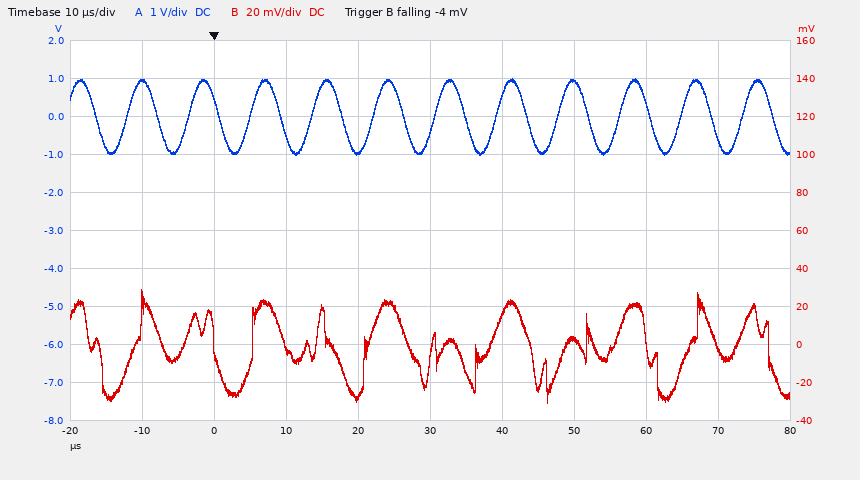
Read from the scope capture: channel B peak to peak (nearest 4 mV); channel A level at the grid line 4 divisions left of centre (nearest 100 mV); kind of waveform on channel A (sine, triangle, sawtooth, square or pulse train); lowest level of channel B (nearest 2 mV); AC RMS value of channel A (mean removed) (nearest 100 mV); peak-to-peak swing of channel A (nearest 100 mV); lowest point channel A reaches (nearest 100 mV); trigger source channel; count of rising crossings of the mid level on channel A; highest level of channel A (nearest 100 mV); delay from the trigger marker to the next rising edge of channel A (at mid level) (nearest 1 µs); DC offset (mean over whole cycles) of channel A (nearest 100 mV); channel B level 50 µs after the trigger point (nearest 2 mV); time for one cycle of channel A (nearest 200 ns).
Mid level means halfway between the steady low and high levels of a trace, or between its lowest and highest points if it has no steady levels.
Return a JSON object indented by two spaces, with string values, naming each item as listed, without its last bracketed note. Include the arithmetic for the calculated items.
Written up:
{
  "channel B peak to peak": "60 mV",
  "channel A level at the grid line 4 divisions left of centre": "900 mV",
  "kind of waveform on channel A": "sine",
  "lowest level of channel B": "-30 mV",
  "AC RMS value of channel A (mean removed)": "2.0 V / (2√2) ≈ 707 mV, so 700 mV to the nearest 100 mV",
  "peak-to-peak swing of channel A": "1.0 V − (-1.0 V) = 2.0 V",
  "lowest point channel A reaches": "-1.0 V",
  "trigger source channel": "channel B",
  "count of rising crossings of the mid level on channel A": "11",
  "highest level of channel A": "1.0 V",
  "delay from the trigger marker to the next rising edge of channel A (at mid level)": "5 µs",
  "DC offset (mean over whole cycles) of channel A": "(1.0 V + (-1.0 V)) / 2 ≈ 0.0 V",
  "channel B level 50 µs after the trigger point": "2 mV",
  "time for one cycle of channel A": "8.6 µs"
}
